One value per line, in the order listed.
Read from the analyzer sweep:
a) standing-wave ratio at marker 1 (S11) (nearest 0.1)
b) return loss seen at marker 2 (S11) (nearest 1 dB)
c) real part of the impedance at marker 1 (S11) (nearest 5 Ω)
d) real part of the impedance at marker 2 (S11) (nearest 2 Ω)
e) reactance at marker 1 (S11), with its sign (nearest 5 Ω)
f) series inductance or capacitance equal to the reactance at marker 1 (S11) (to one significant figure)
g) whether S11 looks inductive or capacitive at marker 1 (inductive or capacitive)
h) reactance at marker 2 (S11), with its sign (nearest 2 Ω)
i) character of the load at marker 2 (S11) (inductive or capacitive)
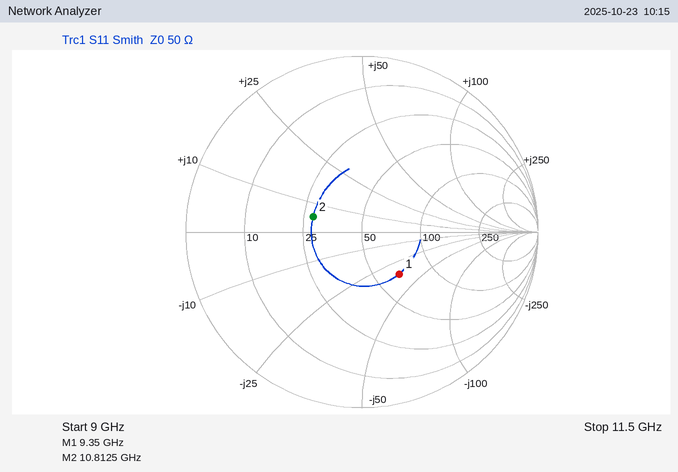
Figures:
1.9
11 dB
65 Ω
28 Ω
-35 Ω
500 fF
capacitive
+6 Ω
inductive
